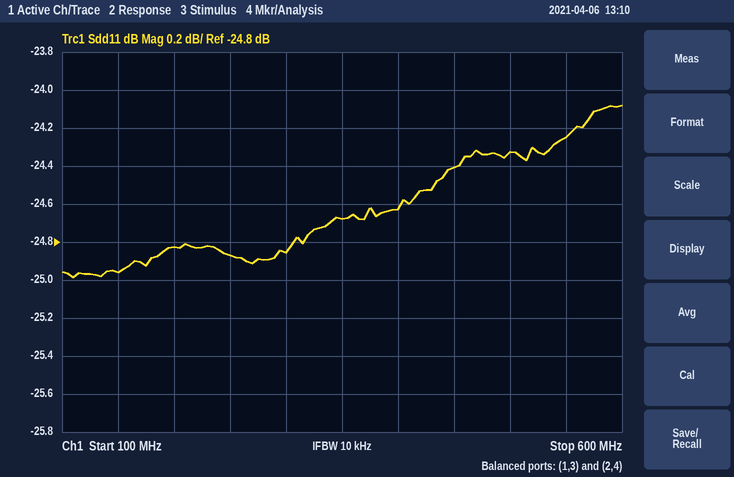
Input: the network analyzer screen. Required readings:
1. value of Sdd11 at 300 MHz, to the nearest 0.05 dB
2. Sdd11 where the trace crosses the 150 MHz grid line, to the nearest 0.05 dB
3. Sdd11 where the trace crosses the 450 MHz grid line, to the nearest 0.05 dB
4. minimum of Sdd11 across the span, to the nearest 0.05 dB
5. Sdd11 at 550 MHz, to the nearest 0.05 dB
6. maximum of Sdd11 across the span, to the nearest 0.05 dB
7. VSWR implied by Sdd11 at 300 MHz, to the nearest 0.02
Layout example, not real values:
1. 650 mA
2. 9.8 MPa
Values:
1. -24.85 dB
2. -24.95 dB
3. -24.40 dB
4. -25.00 dB
5. -24.25 dB
6. -24.10 dB
7. 1.12
